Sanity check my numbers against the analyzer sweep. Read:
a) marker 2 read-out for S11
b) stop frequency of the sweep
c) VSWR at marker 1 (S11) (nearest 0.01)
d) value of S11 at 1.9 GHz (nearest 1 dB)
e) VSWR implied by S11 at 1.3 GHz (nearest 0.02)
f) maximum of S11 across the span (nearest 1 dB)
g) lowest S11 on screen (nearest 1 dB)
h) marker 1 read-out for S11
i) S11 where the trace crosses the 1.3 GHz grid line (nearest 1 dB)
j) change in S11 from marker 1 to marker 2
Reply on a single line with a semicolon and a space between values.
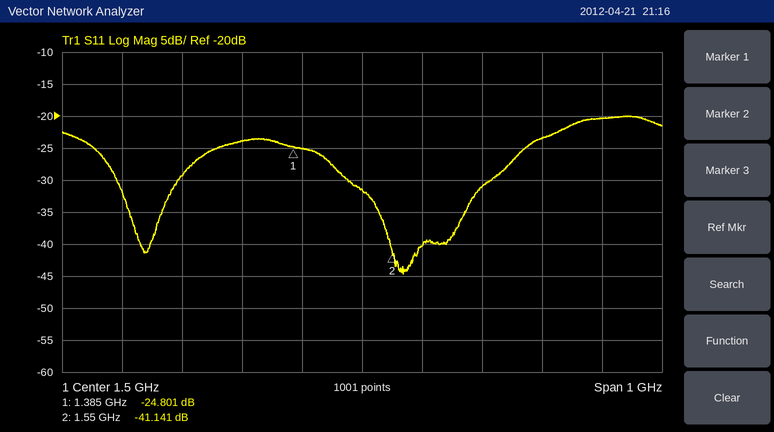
-41.141 dB; 2 GHz; 1.12; -20 dB; 1.14; -20 dB; -45 dB; -24.801 dB; -24 dB; -16.340 dB
